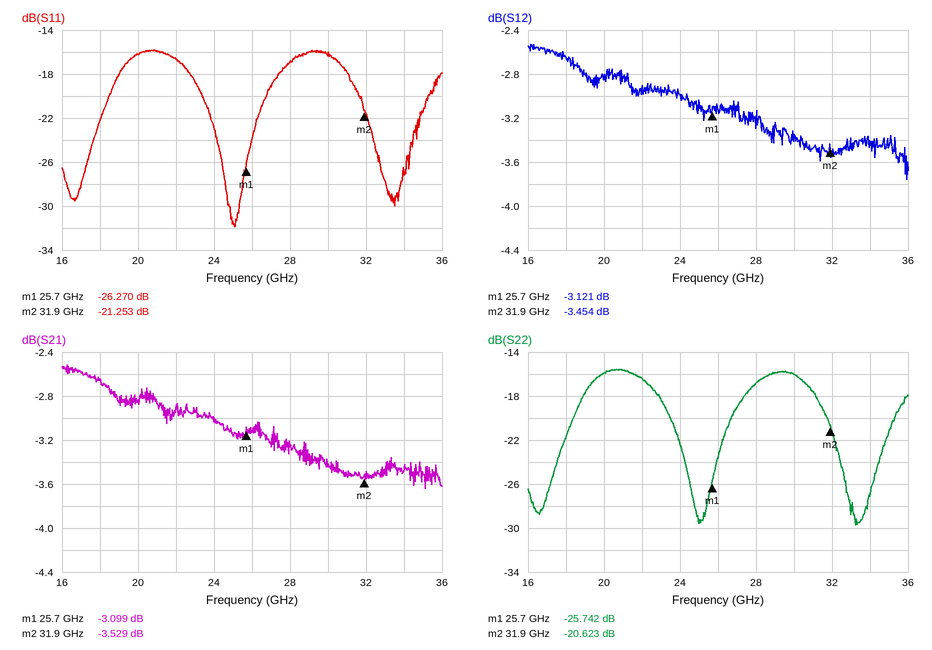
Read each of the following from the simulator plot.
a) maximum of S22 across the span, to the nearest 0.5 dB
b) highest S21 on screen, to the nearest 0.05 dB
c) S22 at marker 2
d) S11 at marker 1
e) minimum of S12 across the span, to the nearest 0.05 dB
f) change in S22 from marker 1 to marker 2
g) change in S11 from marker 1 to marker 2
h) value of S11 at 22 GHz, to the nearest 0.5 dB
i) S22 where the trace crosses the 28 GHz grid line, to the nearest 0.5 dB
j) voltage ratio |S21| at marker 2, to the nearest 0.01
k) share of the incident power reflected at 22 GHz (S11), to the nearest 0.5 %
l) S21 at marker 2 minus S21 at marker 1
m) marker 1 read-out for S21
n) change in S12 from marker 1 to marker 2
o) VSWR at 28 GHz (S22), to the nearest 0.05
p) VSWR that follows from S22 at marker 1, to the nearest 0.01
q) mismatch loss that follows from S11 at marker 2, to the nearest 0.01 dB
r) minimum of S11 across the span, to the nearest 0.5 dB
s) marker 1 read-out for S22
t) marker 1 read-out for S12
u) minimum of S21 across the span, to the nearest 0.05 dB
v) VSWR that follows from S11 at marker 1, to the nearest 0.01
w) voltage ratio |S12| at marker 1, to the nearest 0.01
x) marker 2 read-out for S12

-15.5 dB
-2.50 dB
-20.623 dB
-26.270 dB
-3.75 dB
5.119 dB
5.017 dB
-16.5 dB
-17.0 dB
0.67
2.0 %
-0.430 dB
-3.099 dB
-0.333 dB
1.35
1.11
0.03 dB
-32.0 dB
-25.742 dB
-3.121 dB
-3.65 dB
1.10
0.70
-3.454 dB
